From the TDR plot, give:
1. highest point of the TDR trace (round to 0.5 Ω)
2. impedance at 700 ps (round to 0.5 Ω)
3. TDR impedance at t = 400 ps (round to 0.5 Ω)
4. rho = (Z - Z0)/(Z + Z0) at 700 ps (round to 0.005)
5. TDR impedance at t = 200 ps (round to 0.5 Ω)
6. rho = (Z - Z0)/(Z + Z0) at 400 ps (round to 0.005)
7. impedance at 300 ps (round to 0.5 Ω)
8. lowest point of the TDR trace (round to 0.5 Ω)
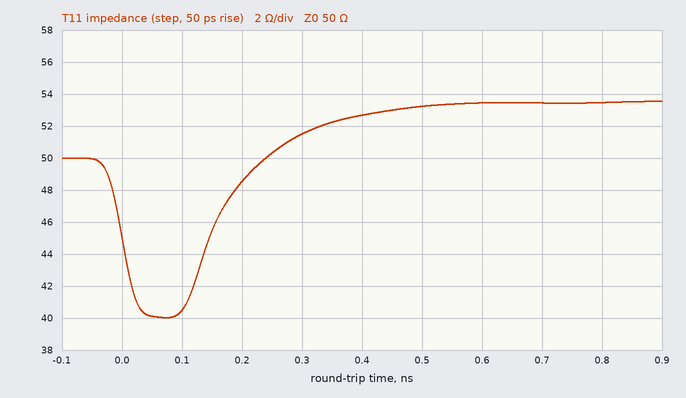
53.5 Ω
53.5 Ω
52.5 Ω
+0.035
48.5 Ω
+0.025
51.5 Ω
40.0 Ω
